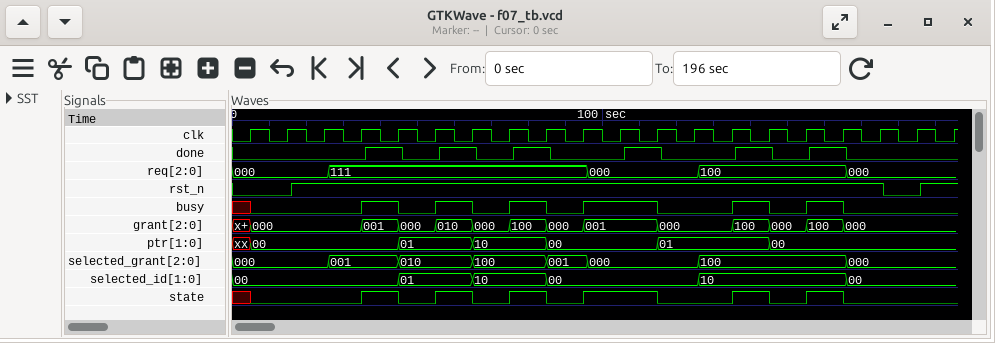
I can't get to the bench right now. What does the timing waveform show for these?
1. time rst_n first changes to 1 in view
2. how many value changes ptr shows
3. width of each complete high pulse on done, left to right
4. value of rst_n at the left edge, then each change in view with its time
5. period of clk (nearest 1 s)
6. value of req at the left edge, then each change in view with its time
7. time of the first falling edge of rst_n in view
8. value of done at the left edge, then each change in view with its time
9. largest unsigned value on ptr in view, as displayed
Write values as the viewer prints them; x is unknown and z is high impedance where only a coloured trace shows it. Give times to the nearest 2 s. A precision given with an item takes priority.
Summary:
16 s
6
10 s, 10 s, 10 s, 10 s, 10 s, 10 s
0, 1 at 16 s, 0 at 176 s, 1 at 186 s
10 s
000, 111 at 26 s, 000 at 96 s, 100 at 126 s, 000 at 166 s
176 s
0, 1 at 36 s, 0 at 46 s, 1 at 56 s, 0 at 66 s, 1 at 76 s, 0 at 86 s, 1 at 106 s, 0 at 116 s, 1 at 136 s, 0 at 146 s, 1 at 156 s, 0 at 166 s
10
